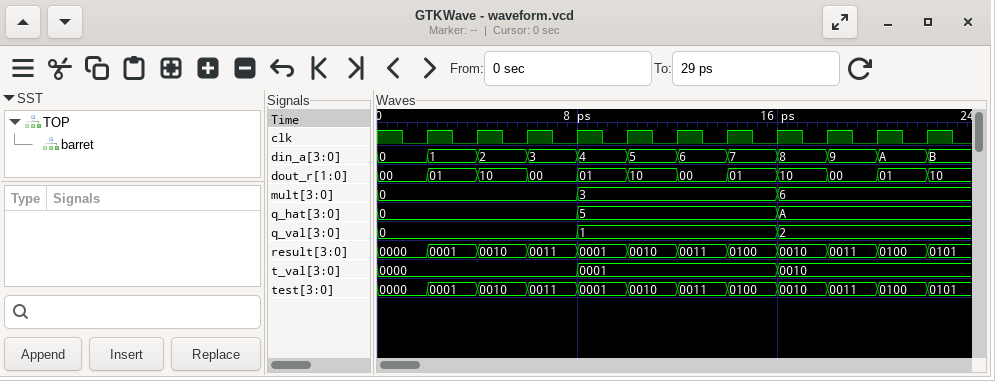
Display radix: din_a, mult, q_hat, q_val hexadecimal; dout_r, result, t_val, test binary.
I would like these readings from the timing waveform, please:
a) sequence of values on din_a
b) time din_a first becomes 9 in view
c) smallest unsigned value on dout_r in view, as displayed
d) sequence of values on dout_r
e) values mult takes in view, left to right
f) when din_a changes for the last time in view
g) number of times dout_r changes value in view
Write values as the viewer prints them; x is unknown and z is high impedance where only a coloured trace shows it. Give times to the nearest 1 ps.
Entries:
0, 1, 2, 3, 4, 5, 6, 7, 8, 9, A, B
18 ps
00
00, 01, 10, 00, 01, 10, 00, 01, 10, 00, 01, 10
0, 3, 6
22 ps
11
